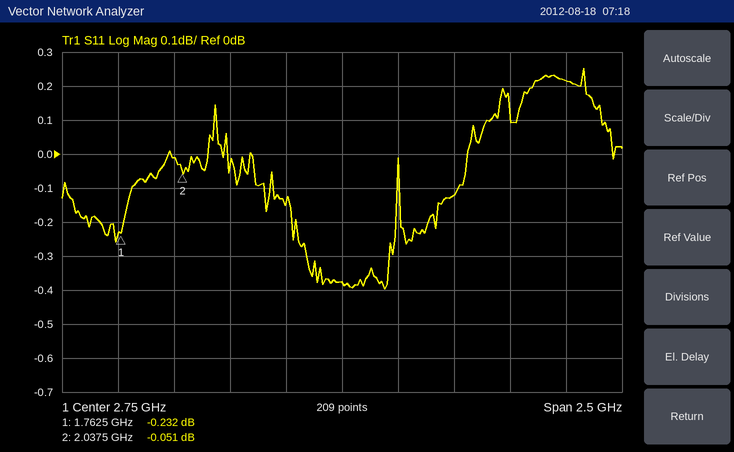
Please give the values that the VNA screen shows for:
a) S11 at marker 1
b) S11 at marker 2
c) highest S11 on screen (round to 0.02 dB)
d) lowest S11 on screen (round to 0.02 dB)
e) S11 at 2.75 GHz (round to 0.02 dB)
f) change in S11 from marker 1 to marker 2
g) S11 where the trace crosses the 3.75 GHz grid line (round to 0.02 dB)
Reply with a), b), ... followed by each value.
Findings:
a) -0.232 dB
b) -0.051 dB
c) 0.26 dB
d) -0.40 dB
e) -0.38 dB
f) 0.181 dB
g) 0.22 dB
